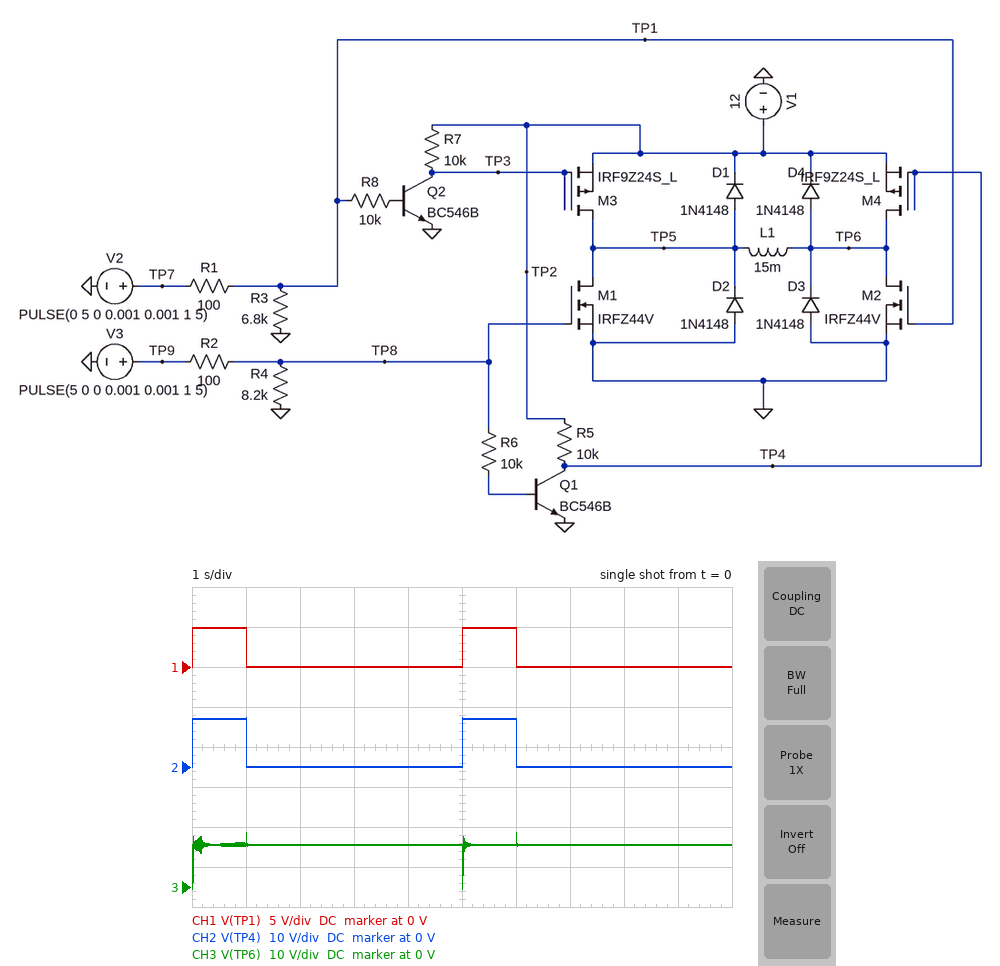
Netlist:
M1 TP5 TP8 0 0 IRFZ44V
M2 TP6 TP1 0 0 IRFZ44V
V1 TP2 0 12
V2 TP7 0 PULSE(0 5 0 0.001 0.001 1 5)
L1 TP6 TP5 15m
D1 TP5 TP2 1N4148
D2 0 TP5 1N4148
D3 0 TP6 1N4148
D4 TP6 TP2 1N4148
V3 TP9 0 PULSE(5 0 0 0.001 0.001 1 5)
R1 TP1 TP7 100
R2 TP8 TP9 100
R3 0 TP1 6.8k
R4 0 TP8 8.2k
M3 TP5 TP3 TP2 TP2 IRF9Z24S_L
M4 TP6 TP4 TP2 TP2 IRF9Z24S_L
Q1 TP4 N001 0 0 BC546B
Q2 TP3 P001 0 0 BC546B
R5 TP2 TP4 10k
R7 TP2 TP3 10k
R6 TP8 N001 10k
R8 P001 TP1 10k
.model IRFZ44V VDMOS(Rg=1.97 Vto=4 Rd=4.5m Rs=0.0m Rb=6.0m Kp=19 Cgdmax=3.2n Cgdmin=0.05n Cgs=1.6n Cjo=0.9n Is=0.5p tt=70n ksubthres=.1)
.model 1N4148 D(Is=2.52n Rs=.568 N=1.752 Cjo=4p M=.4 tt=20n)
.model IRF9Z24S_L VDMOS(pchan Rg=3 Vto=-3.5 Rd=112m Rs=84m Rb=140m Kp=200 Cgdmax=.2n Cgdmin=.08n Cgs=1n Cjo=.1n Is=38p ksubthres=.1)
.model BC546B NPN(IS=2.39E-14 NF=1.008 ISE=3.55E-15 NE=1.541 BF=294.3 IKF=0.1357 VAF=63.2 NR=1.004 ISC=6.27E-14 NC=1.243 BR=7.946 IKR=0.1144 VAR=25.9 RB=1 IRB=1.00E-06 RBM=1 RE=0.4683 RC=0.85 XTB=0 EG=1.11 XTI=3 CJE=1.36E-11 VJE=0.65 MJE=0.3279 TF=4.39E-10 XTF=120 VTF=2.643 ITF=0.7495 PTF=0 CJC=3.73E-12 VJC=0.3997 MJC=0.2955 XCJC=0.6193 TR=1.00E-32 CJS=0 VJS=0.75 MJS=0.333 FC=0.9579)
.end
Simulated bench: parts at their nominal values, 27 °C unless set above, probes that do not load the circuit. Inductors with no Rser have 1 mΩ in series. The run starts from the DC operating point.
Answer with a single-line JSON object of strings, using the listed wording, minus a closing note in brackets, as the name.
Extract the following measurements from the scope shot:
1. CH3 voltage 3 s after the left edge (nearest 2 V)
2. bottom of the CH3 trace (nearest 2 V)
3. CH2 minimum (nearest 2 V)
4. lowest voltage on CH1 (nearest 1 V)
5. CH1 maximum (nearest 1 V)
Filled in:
{"CH3 voltage 3 s after the left edge": "10 V", "bottom of the CH3 trace": "0 V", "CH2 minimum": "0 V", "lowest voltage on CH1": "0 V", "CH1 maximum": "5 V"}
